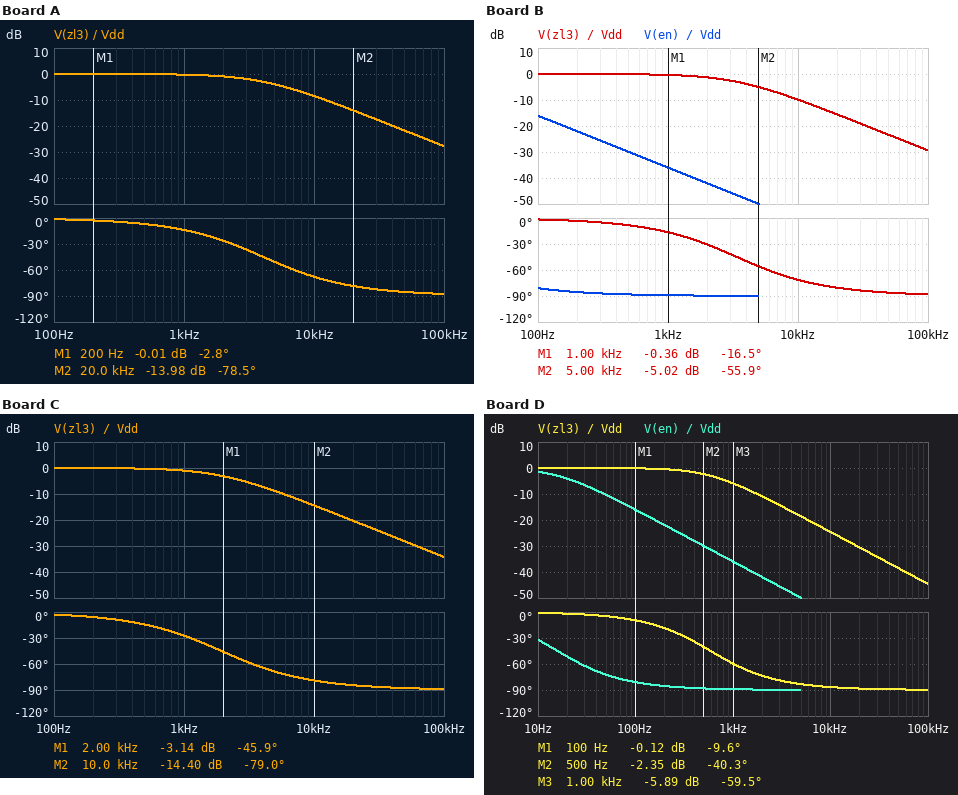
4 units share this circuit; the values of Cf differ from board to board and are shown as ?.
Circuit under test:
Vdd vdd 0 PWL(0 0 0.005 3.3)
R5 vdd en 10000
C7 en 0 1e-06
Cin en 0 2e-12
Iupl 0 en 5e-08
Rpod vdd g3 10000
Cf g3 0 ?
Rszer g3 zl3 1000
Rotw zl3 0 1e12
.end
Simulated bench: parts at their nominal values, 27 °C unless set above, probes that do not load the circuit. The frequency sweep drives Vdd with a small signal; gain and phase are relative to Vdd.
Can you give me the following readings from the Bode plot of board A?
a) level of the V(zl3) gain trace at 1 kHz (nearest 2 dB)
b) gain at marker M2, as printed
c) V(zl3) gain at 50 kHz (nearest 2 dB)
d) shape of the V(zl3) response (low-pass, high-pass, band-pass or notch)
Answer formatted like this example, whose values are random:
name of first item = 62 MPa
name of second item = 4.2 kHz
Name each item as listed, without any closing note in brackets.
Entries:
level of the V(zl3) gain trace at 1 kHz = 0 dB
gain at marker M2, as printed = -13.98 dB
V(zl3) gain at 50 kHz = -22 dB
shape of the V(zl3) response = low-pass
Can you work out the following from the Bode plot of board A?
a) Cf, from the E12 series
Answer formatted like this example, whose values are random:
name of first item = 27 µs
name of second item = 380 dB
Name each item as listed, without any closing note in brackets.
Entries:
Cf, from the E12 series = 3.9 nF
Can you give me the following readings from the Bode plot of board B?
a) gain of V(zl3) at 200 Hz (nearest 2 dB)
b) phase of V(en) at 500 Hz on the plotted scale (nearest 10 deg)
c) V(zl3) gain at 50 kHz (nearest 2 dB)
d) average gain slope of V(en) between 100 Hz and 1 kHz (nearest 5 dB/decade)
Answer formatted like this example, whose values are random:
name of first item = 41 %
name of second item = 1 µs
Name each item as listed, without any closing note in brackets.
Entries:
gain of V(zl3) at 200 Hz = 0 dB
phase of V(en) at 500 Hz on the plotted scale = -90 deg
V(zl3) gain at 50 kHz = -24 dB
average gain slope of V(en) between 100 Hz and 1 kHz = -20 dB/decade
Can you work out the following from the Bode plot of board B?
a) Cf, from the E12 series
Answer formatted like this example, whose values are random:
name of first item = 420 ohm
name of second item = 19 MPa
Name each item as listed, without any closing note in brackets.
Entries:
Cf, from the E12 series = 4.7 nF
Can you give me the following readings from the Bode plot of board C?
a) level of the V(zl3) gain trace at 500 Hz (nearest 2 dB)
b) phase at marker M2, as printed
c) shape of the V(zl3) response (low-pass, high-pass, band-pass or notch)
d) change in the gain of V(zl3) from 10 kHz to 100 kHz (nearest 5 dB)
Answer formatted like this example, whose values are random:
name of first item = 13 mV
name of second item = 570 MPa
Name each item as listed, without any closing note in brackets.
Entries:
level of the V(zl3) gain trace at 500 Hz = 0 dB
phase at marker M2, as printed = -79.0 deg
shape of the V(zl3) response = low-pass
change in the gain of V(zl3) from 10 kHz to 100 kHz = -20 dB
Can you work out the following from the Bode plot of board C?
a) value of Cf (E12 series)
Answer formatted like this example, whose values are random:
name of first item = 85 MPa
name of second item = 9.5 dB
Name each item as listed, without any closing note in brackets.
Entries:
value of Cf = 8.2 nF
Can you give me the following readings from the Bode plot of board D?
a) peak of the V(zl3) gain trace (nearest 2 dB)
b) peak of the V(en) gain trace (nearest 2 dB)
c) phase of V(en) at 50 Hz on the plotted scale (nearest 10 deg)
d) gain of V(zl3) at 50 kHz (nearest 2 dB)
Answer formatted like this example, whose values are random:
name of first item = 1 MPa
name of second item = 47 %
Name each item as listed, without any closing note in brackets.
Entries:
peak of the V(zl3) gain trace = 0 dB
peak of the V(en) gain trace = -2 dB
phase of V(en) at 50 Hz on the plotted scale = -70 deg
gain of V(zl3) at 50 kHz = -38 dB
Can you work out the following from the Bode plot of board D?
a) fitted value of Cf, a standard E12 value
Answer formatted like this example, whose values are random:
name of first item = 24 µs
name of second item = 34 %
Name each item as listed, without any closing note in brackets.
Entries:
fitted value of Cf, a standard E12 value = 27 nF
